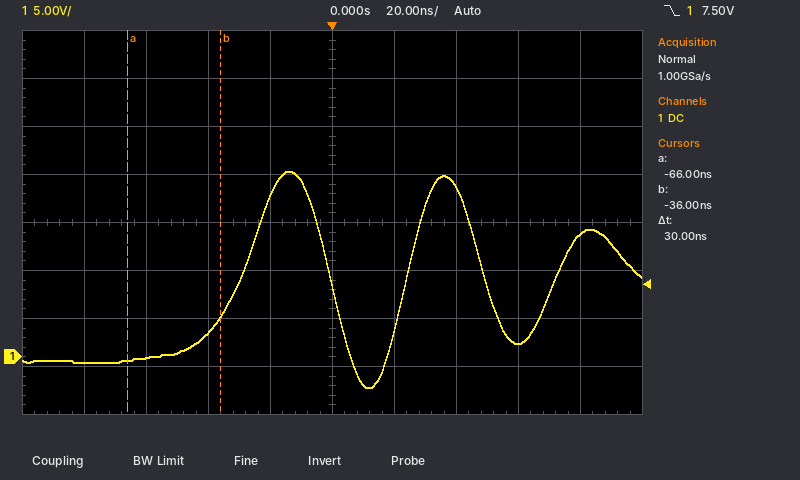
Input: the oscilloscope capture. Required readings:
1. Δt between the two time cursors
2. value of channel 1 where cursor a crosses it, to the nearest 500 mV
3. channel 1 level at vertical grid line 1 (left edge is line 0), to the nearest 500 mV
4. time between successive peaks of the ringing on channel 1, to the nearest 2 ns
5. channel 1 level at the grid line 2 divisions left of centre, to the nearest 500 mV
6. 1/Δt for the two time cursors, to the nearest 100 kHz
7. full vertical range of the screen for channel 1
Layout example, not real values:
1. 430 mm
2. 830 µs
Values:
1. 30 ns
2. -500 mV
3. -500 mV
4. 48 ns
5. 2.5 V
6. 33.3 MHz
7. 40 V
